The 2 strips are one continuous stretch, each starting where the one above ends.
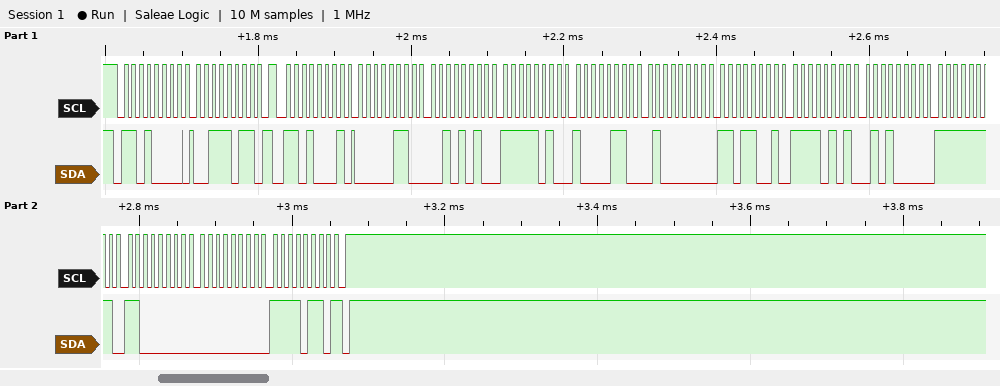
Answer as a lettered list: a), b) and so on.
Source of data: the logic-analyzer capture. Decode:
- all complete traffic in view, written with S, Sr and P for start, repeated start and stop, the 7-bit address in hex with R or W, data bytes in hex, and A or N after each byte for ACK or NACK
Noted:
a) S 68W A 3B A Sr 68R A 06 A 2A A FA A 86 A 40 A D9 A F5 A 50 A FF A C0 A 00 A F6 N P
